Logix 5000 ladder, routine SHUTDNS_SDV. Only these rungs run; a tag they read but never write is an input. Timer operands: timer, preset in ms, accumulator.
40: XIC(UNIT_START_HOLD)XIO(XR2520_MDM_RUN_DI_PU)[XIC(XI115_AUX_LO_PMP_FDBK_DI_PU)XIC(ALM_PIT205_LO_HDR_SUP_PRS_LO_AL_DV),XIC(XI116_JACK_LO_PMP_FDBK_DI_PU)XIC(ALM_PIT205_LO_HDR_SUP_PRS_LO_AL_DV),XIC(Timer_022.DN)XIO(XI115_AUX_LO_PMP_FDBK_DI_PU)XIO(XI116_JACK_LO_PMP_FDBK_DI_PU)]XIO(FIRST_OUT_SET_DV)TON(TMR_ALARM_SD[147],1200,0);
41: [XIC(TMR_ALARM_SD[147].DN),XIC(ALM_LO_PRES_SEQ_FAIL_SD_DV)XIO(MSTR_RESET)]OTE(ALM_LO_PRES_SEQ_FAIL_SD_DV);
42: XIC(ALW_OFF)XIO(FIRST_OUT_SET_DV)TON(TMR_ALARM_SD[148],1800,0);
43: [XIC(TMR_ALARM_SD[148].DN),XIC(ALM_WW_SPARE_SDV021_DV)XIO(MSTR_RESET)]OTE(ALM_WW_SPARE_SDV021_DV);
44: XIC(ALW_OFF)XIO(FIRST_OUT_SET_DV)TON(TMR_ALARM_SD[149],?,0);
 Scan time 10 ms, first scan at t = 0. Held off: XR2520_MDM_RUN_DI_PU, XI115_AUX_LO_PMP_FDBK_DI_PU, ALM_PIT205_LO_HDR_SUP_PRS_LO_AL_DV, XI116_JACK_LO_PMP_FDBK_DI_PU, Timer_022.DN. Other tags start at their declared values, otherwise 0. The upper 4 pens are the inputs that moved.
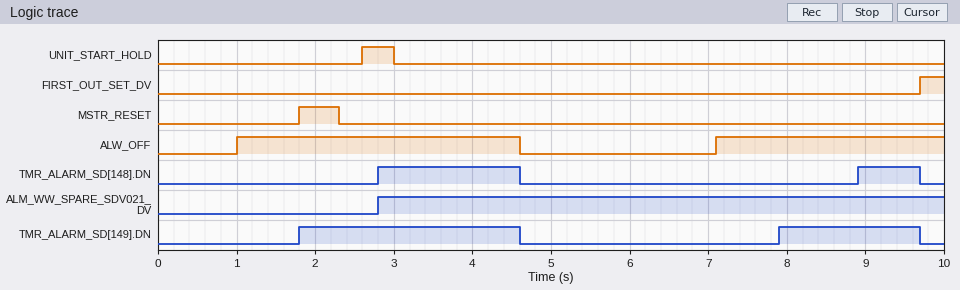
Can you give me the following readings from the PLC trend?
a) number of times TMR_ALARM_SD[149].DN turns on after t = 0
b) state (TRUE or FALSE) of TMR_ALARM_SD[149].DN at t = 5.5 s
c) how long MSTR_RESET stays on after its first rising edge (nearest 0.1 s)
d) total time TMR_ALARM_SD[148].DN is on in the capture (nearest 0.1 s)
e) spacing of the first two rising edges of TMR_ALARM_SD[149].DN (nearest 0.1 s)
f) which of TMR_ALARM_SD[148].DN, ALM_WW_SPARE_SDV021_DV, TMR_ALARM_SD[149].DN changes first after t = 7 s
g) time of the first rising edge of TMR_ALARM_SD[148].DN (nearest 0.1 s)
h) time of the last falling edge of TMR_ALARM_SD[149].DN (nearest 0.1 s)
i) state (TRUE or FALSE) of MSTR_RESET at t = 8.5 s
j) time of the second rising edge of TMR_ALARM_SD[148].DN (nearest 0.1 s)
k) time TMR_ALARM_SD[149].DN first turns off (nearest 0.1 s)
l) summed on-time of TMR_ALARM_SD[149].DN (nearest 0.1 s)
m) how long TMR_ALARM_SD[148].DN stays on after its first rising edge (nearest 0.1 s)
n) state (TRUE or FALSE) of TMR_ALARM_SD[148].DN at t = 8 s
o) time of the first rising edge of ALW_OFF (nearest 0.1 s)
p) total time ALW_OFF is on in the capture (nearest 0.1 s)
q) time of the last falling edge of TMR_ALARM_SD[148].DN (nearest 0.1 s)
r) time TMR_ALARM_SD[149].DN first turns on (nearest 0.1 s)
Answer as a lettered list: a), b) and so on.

a) 2
b) FALSE
c) 0.5 s
d) 2.6 s
e) 6.1 s
f) TMR_ALARM_SD[149].DN
g) 2.8 s
h) 9.7 s
i) FALSE
j) 8.9 s
k) 4.6 s
l) 4.6 s
m) 1.8 s
n) FALSE
o) 1.0 s
p) 6.5 s
q) 9.7 s
r) 1.8 s
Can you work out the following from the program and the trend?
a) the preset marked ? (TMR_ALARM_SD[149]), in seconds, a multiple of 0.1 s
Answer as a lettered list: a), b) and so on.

a) 0.8 s
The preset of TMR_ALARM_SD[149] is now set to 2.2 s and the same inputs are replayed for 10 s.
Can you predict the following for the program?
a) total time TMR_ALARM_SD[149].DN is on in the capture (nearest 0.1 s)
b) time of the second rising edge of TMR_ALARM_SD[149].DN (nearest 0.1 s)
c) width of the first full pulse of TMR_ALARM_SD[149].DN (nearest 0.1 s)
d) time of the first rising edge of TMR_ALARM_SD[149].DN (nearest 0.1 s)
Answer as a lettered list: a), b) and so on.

a) 1.8 s
b) 9.3 s
c) 1.4 s
d) 3.2 s
